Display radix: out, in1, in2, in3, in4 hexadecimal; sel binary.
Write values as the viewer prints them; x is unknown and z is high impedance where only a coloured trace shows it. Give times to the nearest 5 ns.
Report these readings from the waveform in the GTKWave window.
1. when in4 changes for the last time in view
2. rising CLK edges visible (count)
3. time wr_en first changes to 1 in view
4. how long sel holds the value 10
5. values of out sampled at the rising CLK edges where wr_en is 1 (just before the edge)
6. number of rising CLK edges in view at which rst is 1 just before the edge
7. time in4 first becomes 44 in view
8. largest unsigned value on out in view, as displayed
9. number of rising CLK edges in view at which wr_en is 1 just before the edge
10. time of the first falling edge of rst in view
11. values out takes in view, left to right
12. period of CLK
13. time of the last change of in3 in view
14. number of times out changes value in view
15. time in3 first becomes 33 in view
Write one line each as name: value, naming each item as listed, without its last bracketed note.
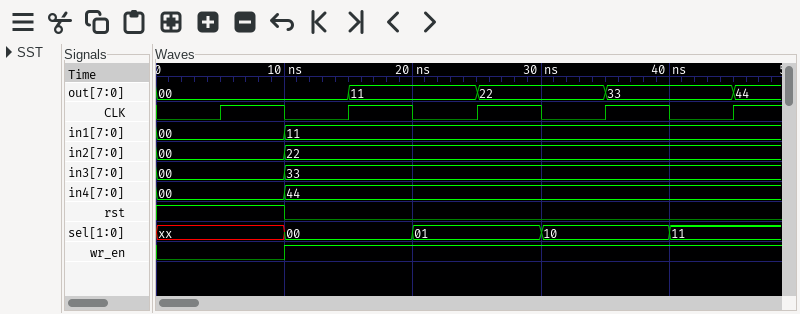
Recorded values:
when in4 changes for the last time in view: 10 ns
rising CLK edges visible: 5
time wr_en first changes to 1 in view: 10 ns
how long sel holds the value 10: 10 ns
values of out sampled at the rising CLK edges where wr_en is 1: 00, 11, 22, 33
number of rising CLK edges in view at which rst is 1 just before the edge: 1
time in4 first becomes 44 in view: 10 ns
largest unsigned value on out in view, as displayed: 44
number of rising CLK edges in view at which wr_en is 1 just before the edge: 4
time of the first falling edge of rst in view: 10 ns
values out takes in view, left to right: 00, 11, 22, 33, 44
period of CLK: 10 ns
time of the last change of in3 in view: 10 ns
number of times out changes value in view: 4
time in3 first becomes 33 in view: 10 ns
